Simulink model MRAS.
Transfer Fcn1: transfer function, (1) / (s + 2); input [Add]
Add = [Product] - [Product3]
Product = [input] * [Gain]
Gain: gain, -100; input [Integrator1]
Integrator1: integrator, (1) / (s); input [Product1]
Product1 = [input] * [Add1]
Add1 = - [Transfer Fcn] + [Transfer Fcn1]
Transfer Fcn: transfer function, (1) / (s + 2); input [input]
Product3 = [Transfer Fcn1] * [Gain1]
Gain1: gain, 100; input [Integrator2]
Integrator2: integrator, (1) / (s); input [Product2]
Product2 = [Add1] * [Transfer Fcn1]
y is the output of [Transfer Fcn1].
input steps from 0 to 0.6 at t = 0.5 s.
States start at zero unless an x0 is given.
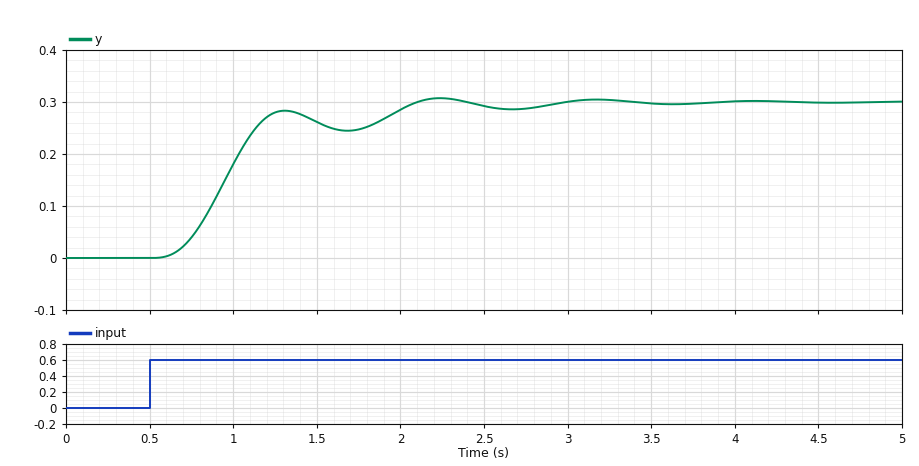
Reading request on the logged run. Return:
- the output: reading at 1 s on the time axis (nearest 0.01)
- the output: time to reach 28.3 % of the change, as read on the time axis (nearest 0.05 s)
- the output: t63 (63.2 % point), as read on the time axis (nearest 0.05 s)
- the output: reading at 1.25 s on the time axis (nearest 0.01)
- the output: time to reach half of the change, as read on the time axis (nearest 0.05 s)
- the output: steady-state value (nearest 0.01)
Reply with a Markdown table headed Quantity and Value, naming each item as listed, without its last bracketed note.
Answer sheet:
| Quantity | Value |
|---|---|
| the output: reading at 1 s on the time axis | 0.18 |
| the output: time to reach 28.3 % of the change, as read on the time axis | 0.85 s |
| the output: t63 (63.2 % point), as read on the time axis | 1.00 s |
| the output: reading at 1.25 s on the time axis | 0.28 |
| the output: time to reach half of the change, as read on the time axis | 0.95 s |
| the output: steady-state value | 0.30 |
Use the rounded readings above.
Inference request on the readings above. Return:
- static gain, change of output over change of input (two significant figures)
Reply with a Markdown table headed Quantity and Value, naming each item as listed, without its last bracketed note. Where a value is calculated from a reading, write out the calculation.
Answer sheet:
| Quantity | Value |
|---|---|
| static gain, change of output over change of input | (0.3 - 0) / (0.6 - 0) = 0.50 |
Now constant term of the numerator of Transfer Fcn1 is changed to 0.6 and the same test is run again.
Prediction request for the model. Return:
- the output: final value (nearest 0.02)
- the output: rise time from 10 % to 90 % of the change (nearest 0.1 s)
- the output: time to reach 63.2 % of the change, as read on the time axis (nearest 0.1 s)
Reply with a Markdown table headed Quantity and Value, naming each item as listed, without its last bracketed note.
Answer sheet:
| Quantity | Value |
|---|---|
| the output: final value | 0.30 |
| the output: rise time from 10 % to 90 % of the change | 0.5 s |
| the output: time to reach 63.2 % of the change, as read on the time axis | 1.1 s |
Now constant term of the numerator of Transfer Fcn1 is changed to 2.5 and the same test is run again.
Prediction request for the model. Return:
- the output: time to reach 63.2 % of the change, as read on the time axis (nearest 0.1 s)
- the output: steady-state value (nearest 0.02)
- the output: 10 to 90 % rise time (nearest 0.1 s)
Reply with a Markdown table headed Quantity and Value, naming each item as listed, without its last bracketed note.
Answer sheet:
| Quantity | Value |
|---|---|
| the output: time to reach 63.2 % of the change, as read on the time axis | 0.9 s |
| the output: steady-state value | 0.30 |
| the output: 10 to 90 % rise time | 0.8 s |
